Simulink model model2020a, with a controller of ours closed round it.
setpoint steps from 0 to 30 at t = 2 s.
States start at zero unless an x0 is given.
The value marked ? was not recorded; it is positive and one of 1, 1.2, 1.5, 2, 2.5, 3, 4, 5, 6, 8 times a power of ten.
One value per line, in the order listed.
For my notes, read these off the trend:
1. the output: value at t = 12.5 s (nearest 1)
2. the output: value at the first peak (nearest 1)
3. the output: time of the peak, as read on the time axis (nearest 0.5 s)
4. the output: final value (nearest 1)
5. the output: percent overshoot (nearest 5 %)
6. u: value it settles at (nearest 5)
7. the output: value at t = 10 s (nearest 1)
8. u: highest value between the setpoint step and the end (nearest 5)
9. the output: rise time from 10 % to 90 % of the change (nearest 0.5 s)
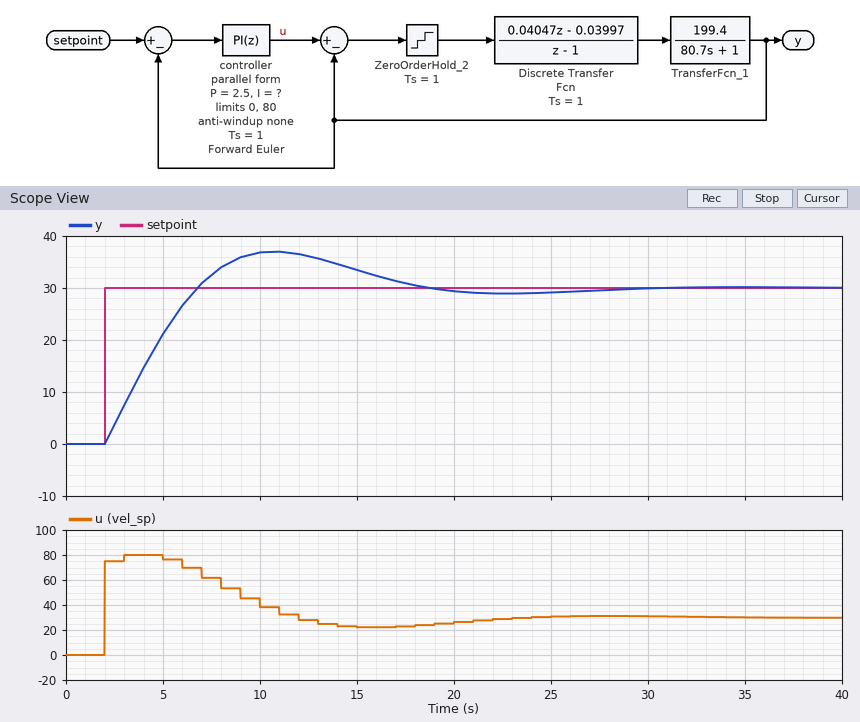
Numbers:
36
37
11.0 s
30
25 %
30
37
80
3.5 s
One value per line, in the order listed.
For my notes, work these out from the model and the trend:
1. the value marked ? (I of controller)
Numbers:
0.8
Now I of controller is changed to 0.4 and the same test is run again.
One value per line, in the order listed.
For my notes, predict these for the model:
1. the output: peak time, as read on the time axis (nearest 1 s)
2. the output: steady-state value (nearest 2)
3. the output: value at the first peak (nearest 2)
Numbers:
15 s
30
32
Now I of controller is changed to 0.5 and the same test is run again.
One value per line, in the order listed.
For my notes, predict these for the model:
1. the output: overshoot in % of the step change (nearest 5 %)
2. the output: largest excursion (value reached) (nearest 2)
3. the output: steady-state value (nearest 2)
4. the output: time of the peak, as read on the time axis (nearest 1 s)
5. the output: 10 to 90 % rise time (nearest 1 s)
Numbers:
10 %
34
30
13 s
5 s
